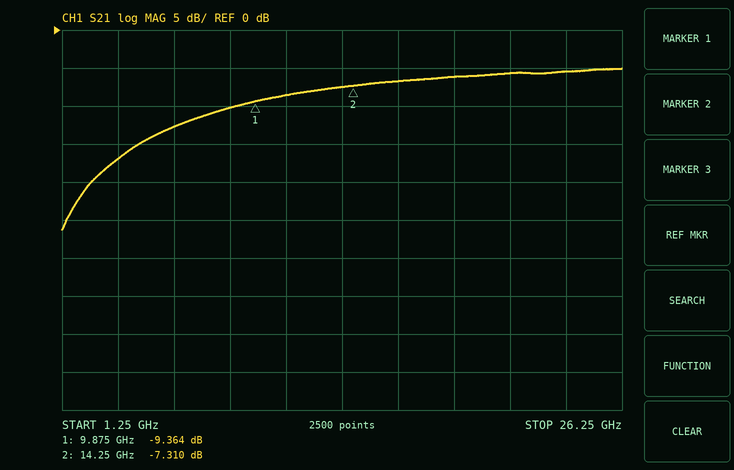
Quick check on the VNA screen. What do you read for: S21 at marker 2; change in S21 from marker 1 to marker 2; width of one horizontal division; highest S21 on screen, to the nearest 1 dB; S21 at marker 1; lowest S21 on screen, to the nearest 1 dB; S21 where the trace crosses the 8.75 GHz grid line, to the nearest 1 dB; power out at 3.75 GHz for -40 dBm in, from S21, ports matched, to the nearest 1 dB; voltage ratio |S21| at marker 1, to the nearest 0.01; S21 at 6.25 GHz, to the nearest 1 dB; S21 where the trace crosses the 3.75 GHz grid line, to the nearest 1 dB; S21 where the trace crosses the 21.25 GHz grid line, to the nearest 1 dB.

-7.310 dB
2.054 dB
2.5 GHz
-5 dB
-9.364 dB
-26 dB
-10 dB
-57 dBm
0.34
-13 dB
-17 dB
-6 dB
